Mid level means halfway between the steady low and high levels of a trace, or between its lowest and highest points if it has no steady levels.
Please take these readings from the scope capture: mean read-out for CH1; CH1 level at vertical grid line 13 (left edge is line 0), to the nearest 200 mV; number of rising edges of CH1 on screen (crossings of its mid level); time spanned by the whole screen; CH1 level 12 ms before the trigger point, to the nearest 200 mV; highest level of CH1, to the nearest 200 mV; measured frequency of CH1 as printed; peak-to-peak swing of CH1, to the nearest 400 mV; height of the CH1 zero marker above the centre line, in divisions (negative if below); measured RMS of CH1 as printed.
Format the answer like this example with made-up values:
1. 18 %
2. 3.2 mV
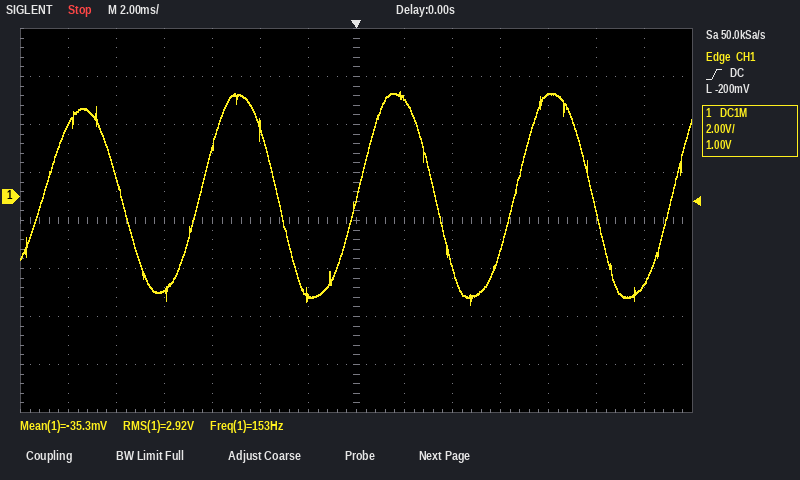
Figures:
1. -35.3 mV
2. -3.6 V
3. 5
4. 28 ms
5. 3.0 V
6. 4.4 V
7. 153 Hz
8. 8.8 V
9. +0.5 div
10. 2.92 V
